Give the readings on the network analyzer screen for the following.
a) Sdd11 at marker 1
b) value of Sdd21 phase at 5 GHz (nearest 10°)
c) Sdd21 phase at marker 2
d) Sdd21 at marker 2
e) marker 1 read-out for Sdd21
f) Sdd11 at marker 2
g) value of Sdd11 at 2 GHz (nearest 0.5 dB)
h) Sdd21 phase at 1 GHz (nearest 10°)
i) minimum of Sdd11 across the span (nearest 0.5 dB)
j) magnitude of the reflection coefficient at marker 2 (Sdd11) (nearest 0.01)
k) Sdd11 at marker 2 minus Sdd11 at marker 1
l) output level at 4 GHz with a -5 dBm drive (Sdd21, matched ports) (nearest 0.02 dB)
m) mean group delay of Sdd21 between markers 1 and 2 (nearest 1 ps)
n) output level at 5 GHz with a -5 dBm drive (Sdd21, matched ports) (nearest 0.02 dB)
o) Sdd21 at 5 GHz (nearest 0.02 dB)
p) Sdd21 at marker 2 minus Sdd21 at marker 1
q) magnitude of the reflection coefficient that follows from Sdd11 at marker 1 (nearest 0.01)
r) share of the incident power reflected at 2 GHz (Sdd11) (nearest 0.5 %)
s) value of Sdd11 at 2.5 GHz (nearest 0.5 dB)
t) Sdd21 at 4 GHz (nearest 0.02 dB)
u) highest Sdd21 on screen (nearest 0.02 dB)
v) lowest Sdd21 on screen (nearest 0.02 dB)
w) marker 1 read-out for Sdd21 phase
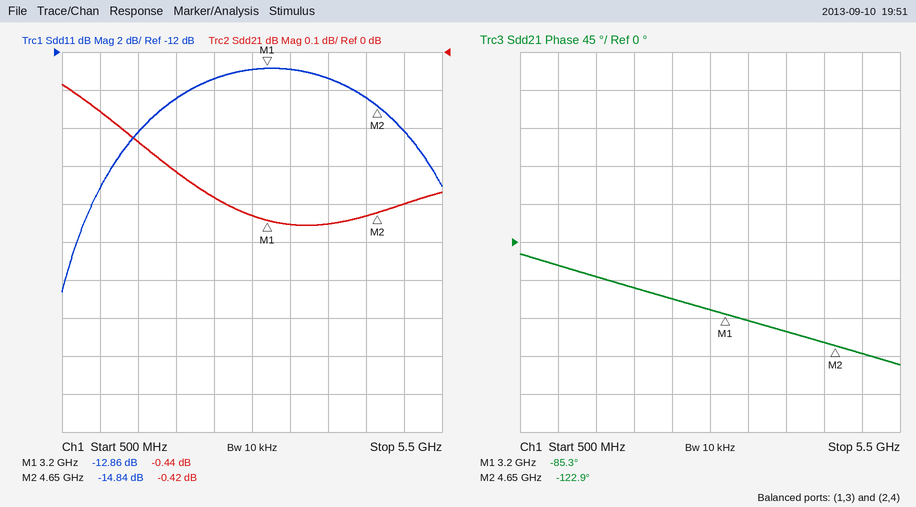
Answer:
-12.86 dB
-130°
-122.9°
-0.42 dB
-0.44 dB
-14.84 dB
-14.5 dB
-30°
-24.5 dB
0.18
-1.98 dB
-5.46 dBm
72 ps
-5.40 dBm
-0.40 dB
0.02 dB
0.23
3.5 %
-13.5 dB
-0.46 dB
-0.08 dB
-0.46 dB
-85.3°
